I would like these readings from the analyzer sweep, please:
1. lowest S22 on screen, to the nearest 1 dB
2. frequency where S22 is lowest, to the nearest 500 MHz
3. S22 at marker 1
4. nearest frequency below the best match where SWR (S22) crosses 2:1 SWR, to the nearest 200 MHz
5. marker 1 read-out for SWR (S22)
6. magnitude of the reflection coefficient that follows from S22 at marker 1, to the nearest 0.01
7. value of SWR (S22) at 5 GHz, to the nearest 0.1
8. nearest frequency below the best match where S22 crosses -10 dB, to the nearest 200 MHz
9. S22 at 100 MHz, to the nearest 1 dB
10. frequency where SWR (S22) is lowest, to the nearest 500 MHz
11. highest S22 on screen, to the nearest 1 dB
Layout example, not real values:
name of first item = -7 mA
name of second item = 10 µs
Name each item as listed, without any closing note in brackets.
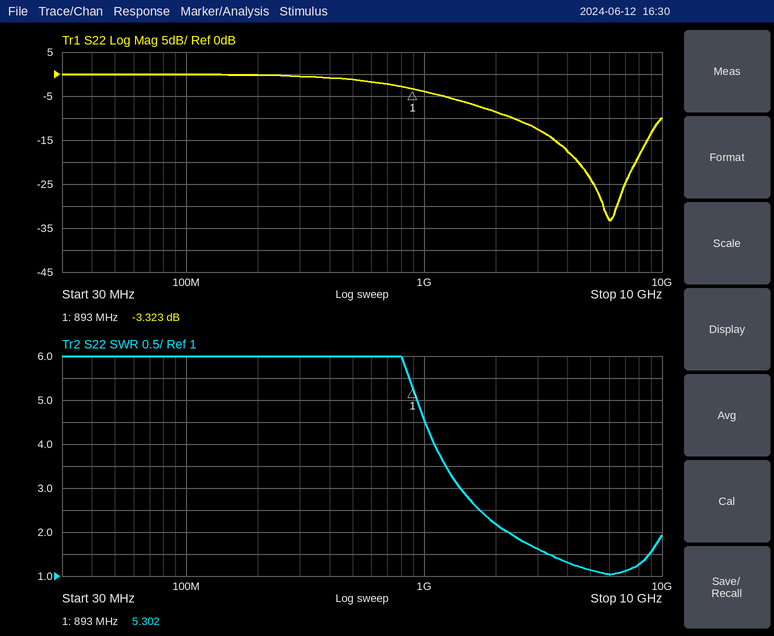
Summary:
lowest S22 on screen, to the nearest 1 dB = -33 dB
frequency where S22 is lowest, to the nearest 500 MHz = 6.0 GHz
S22 at marker 1 = -3.323 dB
nearest frequency below the best match where SWR (S22) crosses 2:1 SWR, to the nearest 200 MHz = 2.2 GHz
marker 1 read-out for SWR = 5.302
magnitude of the reflection coefficient that follows from S22 at marker 1, to the nearest 0.01 = 0.68
value of SWR (S22) at 5 GHz, to the nearest 0.1 = 1.1
nearest frequency below the best match where S22 crosses -10 dB, to the nearest 200 MHz = 2.4 GHz
S22 at 100 MHz, to the nearest 1 dB = 0 dB
frequency where SWR (S22) is lowest, to the nearest 500 MHz = 6.0 GHz
highest S22 on screen, to the nearest 1 dB = 0 dB
